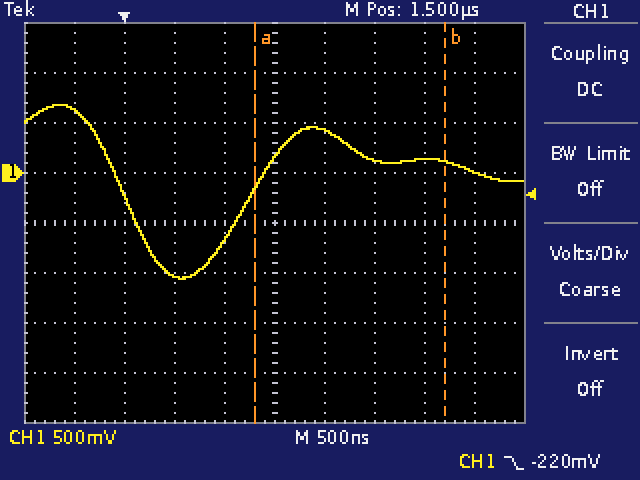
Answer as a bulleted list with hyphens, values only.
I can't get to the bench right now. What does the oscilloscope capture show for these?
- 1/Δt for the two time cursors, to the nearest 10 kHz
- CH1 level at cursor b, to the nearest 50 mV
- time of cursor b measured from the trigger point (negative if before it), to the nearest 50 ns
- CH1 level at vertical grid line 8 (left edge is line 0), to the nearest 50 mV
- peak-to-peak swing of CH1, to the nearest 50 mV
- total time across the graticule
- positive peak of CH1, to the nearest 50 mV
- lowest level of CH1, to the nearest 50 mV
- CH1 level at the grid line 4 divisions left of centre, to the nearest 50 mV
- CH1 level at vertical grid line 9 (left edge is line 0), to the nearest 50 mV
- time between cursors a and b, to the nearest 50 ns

- 530 kHz
- 100 mV
- +3.20 µs
- 150 mV
- 1.75 V
- 5 µs
- 700 mV
- -1.05 V
- 650 mV
- 0 mV
- 1.90 µs
